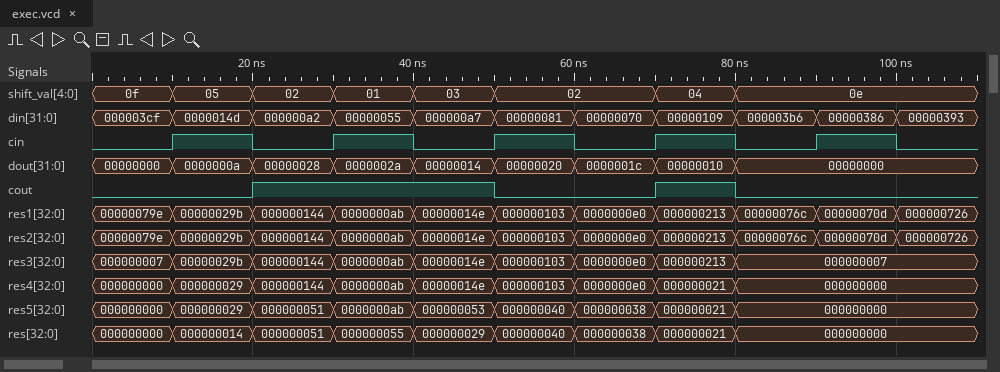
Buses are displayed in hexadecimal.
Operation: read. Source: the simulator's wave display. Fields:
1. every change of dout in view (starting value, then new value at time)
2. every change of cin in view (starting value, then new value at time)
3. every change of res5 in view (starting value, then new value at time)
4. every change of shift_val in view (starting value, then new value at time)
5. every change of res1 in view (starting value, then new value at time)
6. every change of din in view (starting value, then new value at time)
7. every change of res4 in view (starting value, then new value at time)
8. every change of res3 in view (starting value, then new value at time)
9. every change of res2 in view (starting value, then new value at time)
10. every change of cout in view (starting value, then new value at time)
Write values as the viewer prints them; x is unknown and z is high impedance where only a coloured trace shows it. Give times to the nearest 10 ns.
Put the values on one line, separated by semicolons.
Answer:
00000000, 0000000a at 10 ns, 00000028 at 20 ns, 0000002a at 30 ns, 00000014 at 40 ns, 00000020 at 50 ns, 0000001c at 60 ns, 00000010 at 70 ns, 00000000 at 80 ns; 0, 1 at 10 ns, 0 at 20 ns, 1 at 30 ns, 0 at 40 ns, 1 at 50 ns, 0 at 60 ns, 1 at 70 ns, 0 at 80 ns, 1 at 90 ns, 0 at 100 ns; 000000000, 000000029 at 10 ns, 000000051 at 20 ns, 0000000ab at 30 ns, 000000053 at 40 ns, 000000040 at 50 ns, 000000038 at 60 ns, 000000021 at 70 ns, 000000000 at 80 ns; 0f, 05 at 10 ns, 02 at 20 ns, 01 at 30 ns, 03 at 40 ns, 02 at 50 ns, 04 at 70 ns, 0e at 80 ns; 00000079e, 00000029b at 10 ns, 000000144 at 20 ns, 0000000ab at 30 ns, 00000014e at 40 ns, 000000103 at 50 ns, 0000000e0 at 60 ns, 000000213 at 70 ns, 00000076c at 80 ns, 00000070d at 90 ns, 000000726 at 100 ns; 000003cf, 0000014d at 10 ns, 000000a2 at 20 ns, 00000055 at 30 ns, 000000a7 at 40 ns, 00000081 at 50 ns, 00000070 at 60 ns, 00000109 at 70 ns, 000003b6 at 80 ns, 00000386 at 90 ns, 00000393 at 100 ns; 000000000, 000000029 at 10 ns, 000000144 at 20 ns, 0000000ab at 30 ns, 00000014e at 40 ns, 000000103 at 50 ns, 0000000e0 at 60 ns, 000000021 at 70 ns, 000000000 at 80 ns; 000000007, 00000029b at 10 ns, 000000144 at 20 ns, 0000000ab at 30 ns, 00000014e at 40 ns, 000000103 at 50 ns, 0000000e0 at 60 ns, 000000213 at 70 ns, 000000007 at 80 ns; 00000079e, 00000029b at 10 ns, 000000144 at 20 ns, 0000000ab at 30 ns, 00000014e at 40 ns, 000000103 at 50 ns, 0000000e0 at 60 ns, 000000213 at 70 ns, 00000076c at 80 ns, 00000070d at 90 ns, 000000726 at 100 ns; 0, 1 at 20 ns, 0 at 50 ns, 1 at 70 ns, 0 at 80 ns
